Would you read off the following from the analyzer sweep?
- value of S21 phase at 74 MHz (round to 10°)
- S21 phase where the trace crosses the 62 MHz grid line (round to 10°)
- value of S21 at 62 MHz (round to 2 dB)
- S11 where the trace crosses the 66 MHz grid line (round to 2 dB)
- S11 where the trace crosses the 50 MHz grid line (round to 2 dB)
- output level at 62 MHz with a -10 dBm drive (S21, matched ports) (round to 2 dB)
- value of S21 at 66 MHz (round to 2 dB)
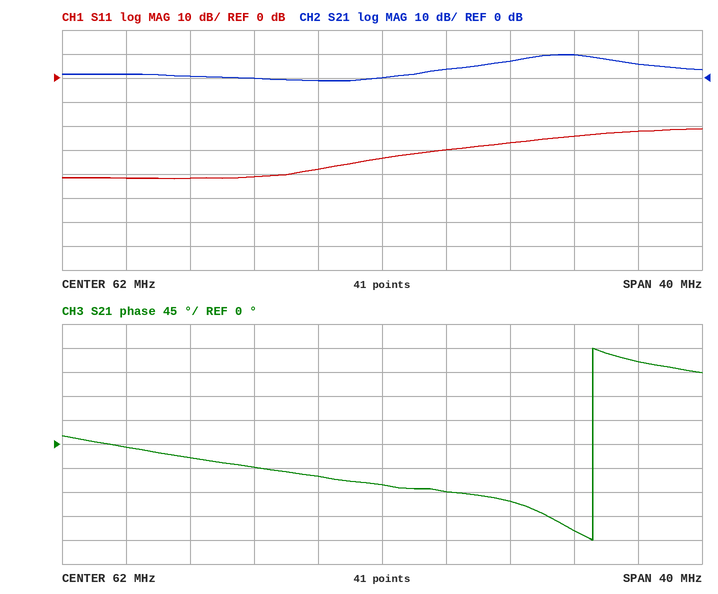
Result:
-160°
-80°
0 dB
-30 dB
-42 dB
-10 dBm
4 dB
